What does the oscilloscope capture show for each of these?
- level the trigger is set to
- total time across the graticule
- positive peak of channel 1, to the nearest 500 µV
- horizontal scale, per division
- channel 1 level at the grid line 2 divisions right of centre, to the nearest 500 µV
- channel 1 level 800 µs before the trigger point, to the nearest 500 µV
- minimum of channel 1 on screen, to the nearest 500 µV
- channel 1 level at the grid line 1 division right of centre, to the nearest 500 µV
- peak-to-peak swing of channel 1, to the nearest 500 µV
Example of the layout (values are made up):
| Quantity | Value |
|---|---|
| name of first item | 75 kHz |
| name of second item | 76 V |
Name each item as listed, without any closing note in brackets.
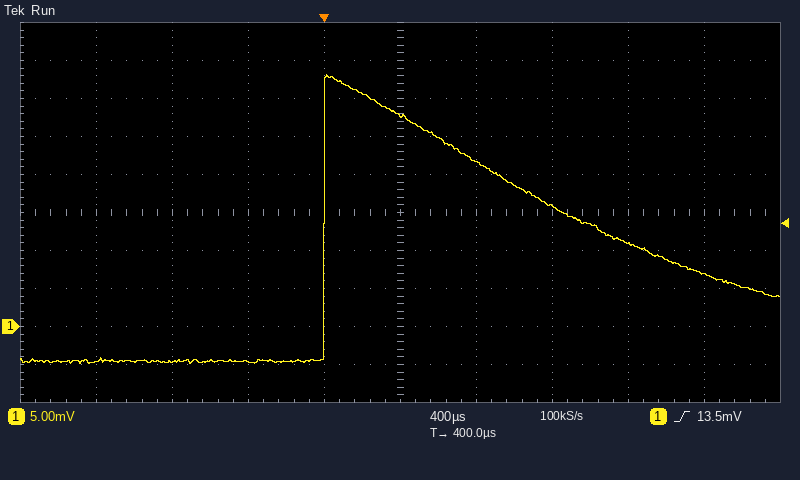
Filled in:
| Quantity | Value |
|---|---|
| level the trigger is set to | 13.5 mV |
| total time across the graticule | 4 ms |
| positive peak of channel 1, to the nearest 500 µV | 33.0 mV |
| horizontal scale, per division | 400 µs |
| channel 1 level at the grid line 2 divisions right of centre, to the nearest 500 µV | 16.0 mV |
| channel 1 level 800 µs before the trigger point, to the nearest 500 µV | -4.5 mV |
| minimum of channel 1 on screen, to the nearest 500 µV | -5.0 mV |
| channel 1 level at the grid line 1 division right of centre, to the nearest 500 µV | 21.5 mV |
| peak-to-peak swing of channel 1, to the nearest 500 µV | 38.0 mV |
